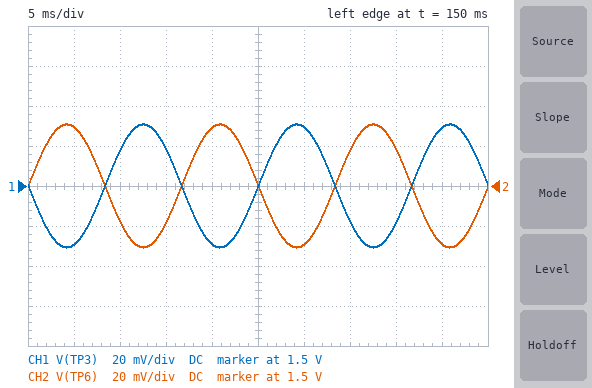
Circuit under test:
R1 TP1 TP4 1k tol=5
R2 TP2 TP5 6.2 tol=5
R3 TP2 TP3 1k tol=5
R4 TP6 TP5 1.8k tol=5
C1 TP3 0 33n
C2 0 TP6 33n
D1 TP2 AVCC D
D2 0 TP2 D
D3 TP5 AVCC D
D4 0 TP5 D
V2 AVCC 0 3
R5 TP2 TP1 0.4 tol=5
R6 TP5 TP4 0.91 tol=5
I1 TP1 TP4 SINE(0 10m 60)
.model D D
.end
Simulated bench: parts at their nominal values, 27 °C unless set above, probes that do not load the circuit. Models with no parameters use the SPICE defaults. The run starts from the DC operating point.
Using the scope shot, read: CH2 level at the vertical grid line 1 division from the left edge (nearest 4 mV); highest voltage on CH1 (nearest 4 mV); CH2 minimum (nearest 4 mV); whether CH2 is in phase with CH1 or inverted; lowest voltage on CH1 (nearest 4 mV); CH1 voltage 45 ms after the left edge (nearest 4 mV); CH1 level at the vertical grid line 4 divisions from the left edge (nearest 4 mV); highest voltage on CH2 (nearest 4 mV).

1.528 V
1.532 V
1.468 V
inverted
1.468 V
1.528 V
1.472 V
1.532 V
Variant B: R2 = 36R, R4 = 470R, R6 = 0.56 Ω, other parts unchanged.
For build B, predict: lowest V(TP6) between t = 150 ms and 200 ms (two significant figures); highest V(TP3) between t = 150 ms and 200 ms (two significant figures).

1.3 V
1.7 V
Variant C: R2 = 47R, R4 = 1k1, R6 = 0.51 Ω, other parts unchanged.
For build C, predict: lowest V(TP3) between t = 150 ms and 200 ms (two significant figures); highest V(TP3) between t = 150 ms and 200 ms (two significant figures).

1.3 V
1.7 V
